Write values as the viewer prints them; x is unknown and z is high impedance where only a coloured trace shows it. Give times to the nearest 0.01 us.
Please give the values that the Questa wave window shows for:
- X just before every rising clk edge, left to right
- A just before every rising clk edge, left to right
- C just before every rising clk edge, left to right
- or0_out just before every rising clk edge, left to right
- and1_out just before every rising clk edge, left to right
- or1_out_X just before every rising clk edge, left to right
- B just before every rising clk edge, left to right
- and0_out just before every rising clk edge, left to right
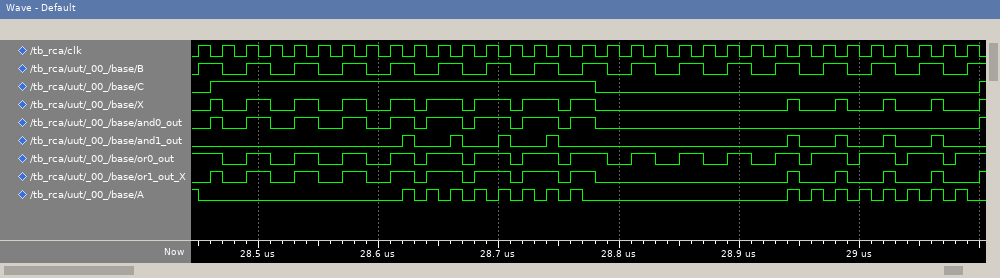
0 1 0 1 0 1 0 1 0 1 1 1 1 1 1 1 1 0 0 0 0 0 0 0 0 1 0 1 0 1 0 1 0
1 0 0 0 0 0 0 0 0 1 1 1 1 1 1 1 1 0 0 0 0 0 0 0 0 1 1 1 1 1 1 1 1
0 1 1 1 1 1 1 1 1 1 1 1 1 1 1 1 1 0 0 0 0 0 0 0 0 0 0 0 0 0 0 0 0
1 1 0 1 0 1 0 1 0 1 1 1 1 1 1 1 1 1 0 1 0 1 0 1 0 1 1 1 1 1 1 1 1
0 0 0 0 0 0 0 0 0 1 0 1 0 1 0 1 0 0 0 0 0 0 0 0 0 1 0 1 0 1 0 1 0
0 1 0 1 0 1 0 1 0 1 1 1 1 1 1 1 1 0 0 0 0 0 0 0 0 1 0 1 0 1 0 1 0
0 1 0 1 0 1 0 1 0 1 0 1 0 1 0 1 0 1 0 1 0 1 0 1 0 1 0 1 0 1 0 1 0
0 1 0 1 0 1 0 1 0 1 1 1 1 1 1 1 1 0 0 0 0 0 0 0 0 0 0 0 0 0 0 0 0
